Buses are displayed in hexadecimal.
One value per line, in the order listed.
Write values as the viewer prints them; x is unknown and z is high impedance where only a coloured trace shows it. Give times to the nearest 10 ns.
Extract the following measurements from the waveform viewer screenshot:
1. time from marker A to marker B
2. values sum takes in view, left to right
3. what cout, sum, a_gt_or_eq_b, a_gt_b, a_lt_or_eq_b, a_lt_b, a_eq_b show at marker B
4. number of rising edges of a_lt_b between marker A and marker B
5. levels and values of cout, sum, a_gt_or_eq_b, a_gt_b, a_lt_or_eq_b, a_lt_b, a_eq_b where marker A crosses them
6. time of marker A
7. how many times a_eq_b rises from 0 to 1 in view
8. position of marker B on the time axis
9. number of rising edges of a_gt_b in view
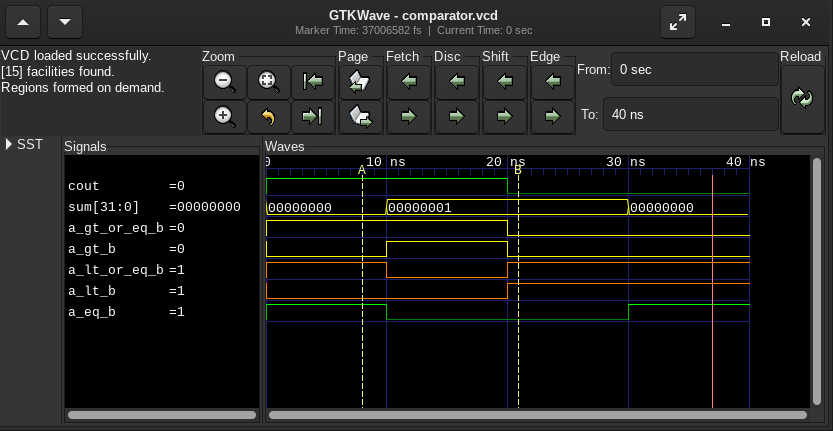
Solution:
10 ns
00000000, 00000001, 00000000
cout=0, sum=00000001, a_gt_or_eq_b=0, a_gt_b=0, a_lt_or_eq_b=1, a_lt_b=1, a_eq_b=0
1
cout=1, sum=00000000, a_gt_or_eq_b=1, a_gt_b=0, a_lt_or_eq_b=1, a_lt_b=0, a_eq_b=1
10 ns
1
20 ns
1
